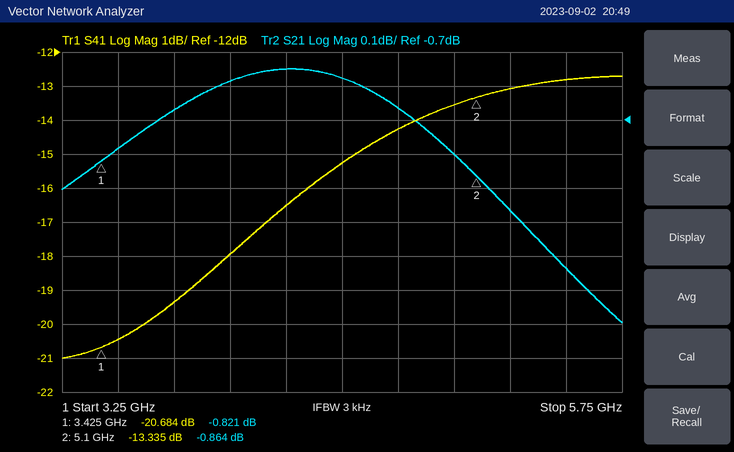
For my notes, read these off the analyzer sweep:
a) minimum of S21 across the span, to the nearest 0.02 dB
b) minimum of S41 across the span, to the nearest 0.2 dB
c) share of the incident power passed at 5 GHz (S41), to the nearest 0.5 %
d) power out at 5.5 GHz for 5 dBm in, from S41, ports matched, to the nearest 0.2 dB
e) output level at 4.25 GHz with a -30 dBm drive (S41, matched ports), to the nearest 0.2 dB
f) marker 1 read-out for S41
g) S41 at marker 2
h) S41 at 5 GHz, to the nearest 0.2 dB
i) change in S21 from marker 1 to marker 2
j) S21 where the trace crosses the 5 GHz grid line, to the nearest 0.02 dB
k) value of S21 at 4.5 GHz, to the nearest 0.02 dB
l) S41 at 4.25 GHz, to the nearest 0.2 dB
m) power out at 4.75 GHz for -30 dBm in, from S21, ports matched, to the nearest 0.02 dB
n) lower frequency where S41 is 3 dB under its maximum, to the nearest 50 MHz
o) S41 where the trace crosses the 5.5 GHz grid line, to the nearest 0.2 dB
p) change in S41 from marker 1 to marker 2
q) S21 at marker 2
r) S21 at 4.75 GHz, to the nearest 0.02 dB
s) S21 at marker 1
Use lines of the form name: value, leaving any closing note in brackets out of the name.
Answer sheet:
minimum of S21 across the span, to the nearest 0.02 dB: -1.30 dB
minimum of S41 across the span, to the nearest 0.2 dB: -21.0 dB
share of the incident power passed at 5 GHz (S41), to the nearest 0.5 %: 4.5 %
power out at 5.5 GHz for 5 dBm in, from S41, ports matched, to the nearest 0.2 dB: -7.8 dBm
output level at 4.25 GHz with a -30 dBm drive (S41, matched ports), to the nearest 0.2 dB: -46.6 dBm
marker 1 read-out for S41: -20.684 dB
S41 at marker 2: -13.335 dB
S41 at 5 GHz, to the nearest 0.2 dB: -13.6 dB
change in S21 from marker 1 to marker 2: -0.043 dB
S21 where the trace crosses the 5 GHz grid line, to the nearest 0.02 dB: -0.80 dB
value of S21 at 4.5 GHz, to the nearest 0.02 dB: -0.58 dB
S41 at 4.25 GHz, to the nearest 0.2 dB: -16.6 dB
power out at 4.75 GHz for -30 dBm in, from S21, ports matched, to the nearest 0.02 dB: -30.66 dBm
lower frequency where S41 is 3 dB under its maximum, to the nearest 50 MHz: 4.40 GHz
S41 where the trace crosses the 5.5 GHz grid line, to the nearest 0.2 dB: -12.8 dB
change in S41 from marker 1 to marker 2: 7.349 dB
S21 at marker 2: -0.864 dB
S21 at 4.75 GHz, to the nearest 0.02 dB: -0.66 dB
S21 at marker 1: -0.821 dB
